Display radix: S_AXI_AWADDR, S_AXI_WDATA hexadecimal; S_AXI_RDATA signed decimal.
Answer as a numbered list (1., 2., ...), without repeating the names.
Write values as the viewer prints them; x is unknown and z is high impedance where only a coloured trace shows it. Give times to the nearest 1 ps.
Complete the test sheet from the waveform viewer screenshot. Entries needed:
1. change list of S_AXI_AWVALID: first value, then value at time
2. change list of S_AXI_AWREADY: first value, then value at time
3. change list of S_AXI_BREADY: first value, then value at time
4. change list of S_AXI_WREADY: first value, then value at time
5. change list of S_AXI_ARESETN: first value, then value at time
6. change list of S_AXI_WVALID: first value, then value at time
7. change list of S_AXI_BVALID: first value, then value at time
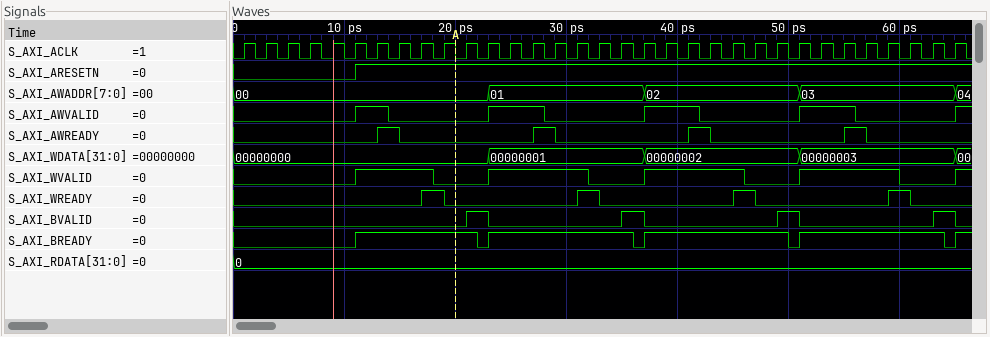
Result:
1. 0, 1 at 11 ps, 0 at 14 ps, 1 at 23 ps, 0 at 28 ps, 1 at 37 ps, 0 at 42 ps, 1 at 51 ps, 0 at 56 ps, 1 at 65 ps
2. 0, 1 at 13 ps, 0 at 15 ps, 1 at 27 ps, 0 at 29 ps, 1 at 41 ps, 0 at 43 ps, 1 at 55 ps, 0 at 57 ps
3. 0, 1 at 11 ps, 0 at 22 ps, 1 at 23 ps, 0 at 36 ps, 1 at 37 ps, 0 at 50 ps, 1 at 51 ps, 0 at 64 ps, 1 at 65 ps
4. 0, 1 at 17 ps, 0 at 19 ps, 1 at 31 ps, 0 at 33 ps, 1 at 45 ps, 0 at 47 ps, 1 at 59 ps, 0 at 61 ps
5. 0, 1 at 11 ps
6. 0, 1 at 11 ps, 0 at 18 ps, 1 at 23 ps, 0 at 32 ps, 1 at 37 ps, 0 at 46 ps, 1 at 51 ps, 0 at 60 ps, 1 at 65 ps
7. 0, 1 at 21 ps, 0 at 23 ps, 1 at 35 ps, 0 at 37 ps, 1 at 49 ps, 0 at 51 ps, 1 at 63 ps, 0 at 65 ps
